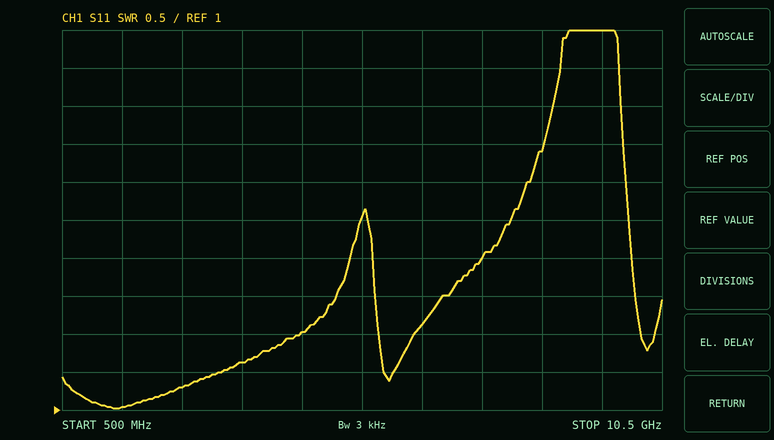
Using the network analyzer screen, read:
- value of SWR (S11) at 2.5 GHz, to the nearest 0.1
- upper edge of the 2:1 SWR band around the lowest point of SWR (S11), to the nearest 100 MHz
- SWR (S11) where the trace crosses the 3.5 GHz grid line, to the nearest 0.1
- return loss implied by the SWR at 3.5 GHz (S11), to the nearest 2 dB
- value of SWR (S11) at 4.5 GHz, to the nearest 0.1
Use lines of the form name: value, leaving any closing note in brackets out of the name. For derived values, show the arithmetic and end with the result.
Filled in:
value of SWR (S11) at 2.5 GHz, to the nearest 0.1: 1.3
upper edge of the 2:1 SWR band around the lowest point of SWR (S11), to the nearest 100 MHz: 4.5 GHz
SWR (S11) where the trace crosses the 3.5 GHz grid line, to the nearest 0.1: 1.6
return loss implied by the SWR at 3.5 GHz (S11), to the nearest 2 dB: −20 log10((1.6 − 1)/(1.6 + 1)) ≈ 12.7 dB, so 12 dB to the nearest 2 dB
value of SWR (S11) at 4.5 GHz, to the nearest 0.1: 2.0
